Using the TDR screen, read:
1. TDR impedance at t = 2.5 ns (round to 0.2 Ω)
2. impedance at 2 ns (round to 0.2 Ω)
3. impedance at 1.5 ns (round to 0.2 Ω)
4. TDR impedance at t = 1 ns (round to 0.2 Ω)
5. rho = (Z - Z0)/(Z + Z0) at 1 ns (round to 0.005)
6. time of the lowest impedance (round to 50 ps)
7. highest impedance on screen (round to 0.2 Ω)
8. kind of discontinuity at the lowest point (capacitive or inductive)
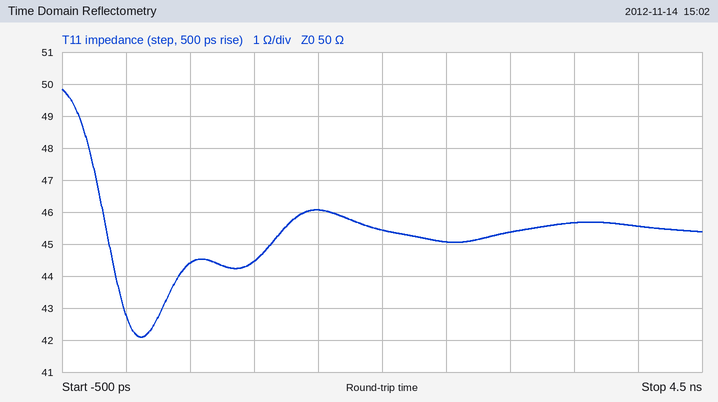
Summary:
45.0 Ω
45.4 Ω
46.0 Ω
44.4 Ω
-0.060
100 ps
49.8 Ω
capacitive
